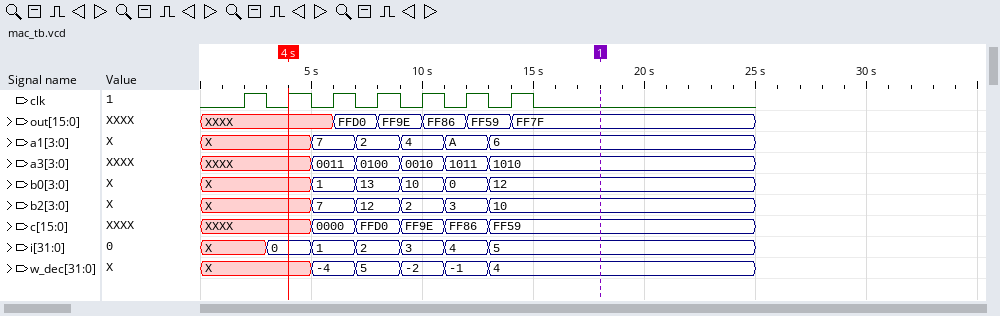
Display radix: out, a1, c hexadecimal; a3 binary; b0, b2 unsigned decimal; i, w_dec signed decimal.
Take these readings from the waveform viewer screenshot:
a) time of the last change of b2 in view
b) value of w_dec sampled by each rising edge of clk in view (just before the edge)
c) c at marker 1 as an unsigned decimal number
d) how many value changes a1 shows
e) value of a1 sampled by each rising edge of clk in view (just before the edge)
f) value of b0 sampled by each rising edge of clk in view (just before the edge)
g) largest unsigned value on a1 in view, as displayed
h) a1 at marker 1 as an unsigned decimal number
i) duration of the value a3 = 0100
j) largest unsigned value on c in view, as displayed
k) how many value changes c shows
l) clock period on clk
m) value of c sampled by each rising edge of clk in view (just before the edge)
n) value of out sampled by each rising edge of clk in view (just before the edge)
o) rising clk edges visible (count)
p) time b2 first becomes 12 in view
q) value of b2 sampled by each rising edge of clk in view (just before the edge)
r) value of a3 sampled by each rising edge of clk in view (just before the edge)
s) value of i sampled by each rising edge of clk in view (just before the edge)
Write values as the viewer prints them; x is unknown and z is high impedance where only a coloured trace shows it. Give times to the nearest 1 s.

13 s
X, X, -4, 5, -2, -1, 4
65369
5
X, X, 7, 2, 4, A, 6
X, X, 1, 13, 10, 0, 12
A
6
2 s
FFD0
5
2 s
XXXX, XXXX, 0000, FFD0, FF9E, FF86, FF59
XXXX, XXXX, XXXX, FFD0, FF9E, FF86, FF59
7
7 s
X, X, 7, 12, 2, 3, 10
XXXX, XXXX, 0011, 0100, 0010, 1011, 1010
X, 0, 1, 2, 3, 4, 5
